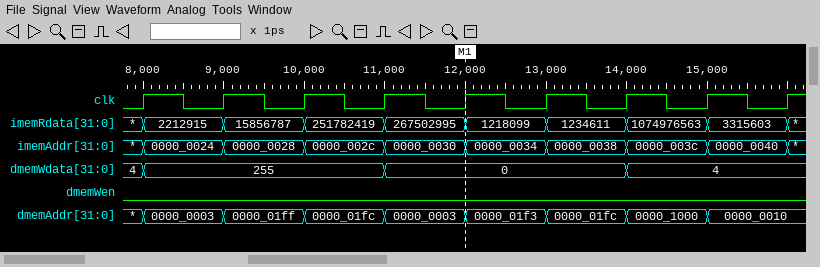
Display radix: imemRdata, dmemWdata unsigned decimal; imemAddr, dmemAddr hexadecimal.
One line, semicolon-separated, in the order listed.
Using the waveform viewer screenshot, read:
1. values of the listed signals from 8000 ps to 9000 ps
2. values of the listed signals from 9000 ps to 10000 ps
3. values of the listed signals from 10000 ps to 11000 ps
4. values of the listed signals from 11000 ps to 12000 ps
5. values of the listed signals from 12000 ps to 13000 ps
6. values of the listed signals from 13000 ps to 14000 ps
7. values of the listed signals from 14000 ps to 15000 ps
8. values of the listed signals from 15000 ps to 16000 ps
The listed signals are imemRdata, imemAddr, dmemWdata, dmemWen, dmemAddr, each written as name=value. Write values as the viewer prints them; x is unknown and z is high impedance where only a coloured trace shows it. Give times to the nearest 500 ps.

imemRdata=2212915, imemAddr=0000_0024, dmemWdata=255, dmemWen=0, dmemAddr=0000_0003; imemRdata=15856787, imemAddr=0000_0028, dmemWdata=255, dmemWen=0, dmemAddr=0000_01ff; imemRdata=251782419, imemAddr=0000_002c, dmemWdata=255, dmemWen=0, dmemAddr=0000_01fc; imemRdata=267502995, imemAddr=0000_0030, dmemWdata=0, dmemWen=0, dmemAddr=0000_0003; imemRdata=1218099, imemAddr=0000_0034, dmemWdata=0, dmemWen=0, dmemAddr=0000_01f3; imemRdata=1234611, imemAddr=0000_0038, dmemWdata=0, dmemWen=0, dmemAddr=0000_01fc; imemRdata=1074976563, imemAddr=0000_003c, dmemWdata=4, dmemWen=0, dmemAddr=0000_1000; imemRdata=3315603, imemAddr=0000_0040, dmemWdata=4, dmemWen=0, dmemAddr=0000_0010
